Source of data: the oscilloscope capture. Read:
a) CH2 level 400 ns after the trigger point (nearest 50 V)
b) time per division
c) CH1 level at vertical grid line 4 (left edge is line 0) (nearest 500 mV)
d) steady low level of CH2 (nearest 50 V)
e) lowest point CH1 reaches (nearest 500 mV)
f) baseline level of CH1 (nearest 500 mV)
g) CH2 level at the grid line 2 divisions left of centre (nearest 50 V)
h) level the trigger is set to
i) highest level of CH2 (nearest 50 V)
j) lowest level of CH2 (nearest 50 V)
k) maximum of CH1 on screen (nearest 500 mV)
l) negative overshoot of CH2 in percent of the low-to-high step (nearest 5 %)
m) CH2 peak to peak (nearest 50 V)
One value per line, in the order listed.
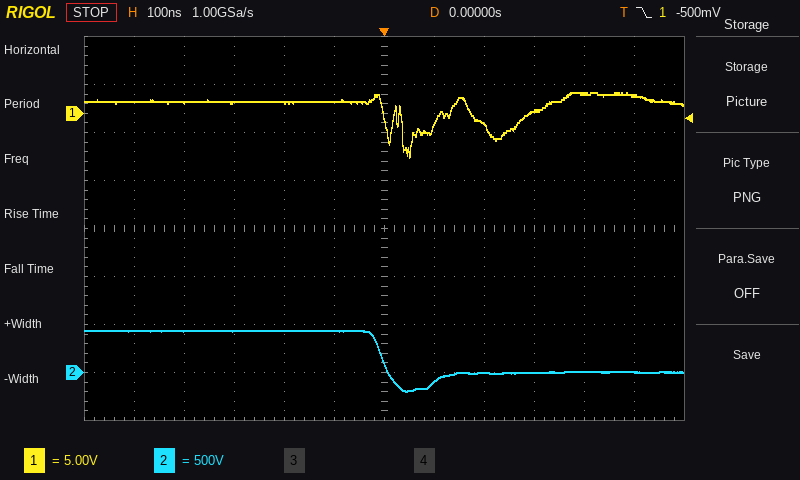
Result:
0 V
100 ns
1.0 V
0 V
-4.5 V
1.0 V
450 V
-500 mV
450 V
-200 V
2.0 V
45 %
650 V
